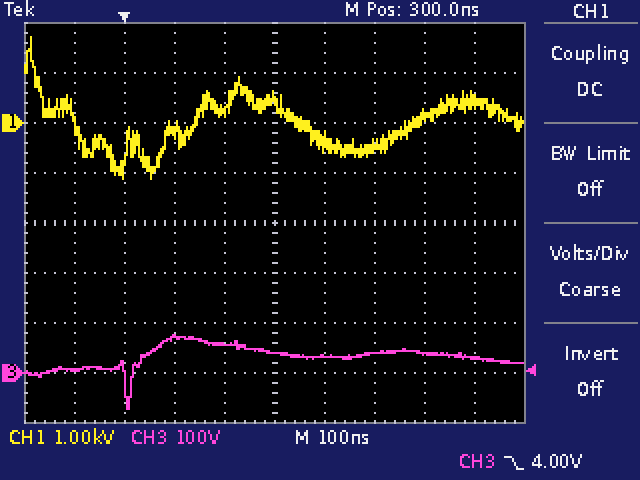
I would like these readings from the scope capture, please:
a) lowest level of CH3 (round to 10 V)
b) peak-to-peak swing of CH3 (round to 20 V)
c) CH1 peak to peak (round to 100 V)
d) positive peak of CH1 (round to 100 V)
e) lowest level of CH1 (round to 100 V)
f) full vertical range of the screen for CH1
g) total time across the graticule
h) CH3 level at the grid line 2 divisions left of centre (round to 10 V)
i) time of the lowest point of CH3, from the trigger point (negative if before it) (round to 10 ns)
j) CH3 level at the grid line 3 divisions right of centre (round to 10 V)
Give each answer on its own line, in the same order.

-70 V
140 V
2.8 kV
1.7 kV
-1.1 kV
8 kV
1 µs
70 V
+10 ns
40 V
